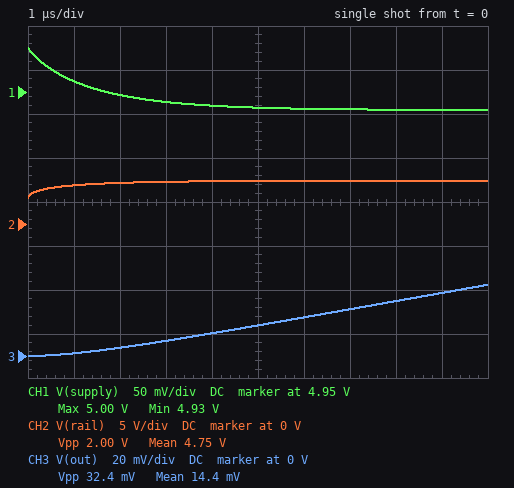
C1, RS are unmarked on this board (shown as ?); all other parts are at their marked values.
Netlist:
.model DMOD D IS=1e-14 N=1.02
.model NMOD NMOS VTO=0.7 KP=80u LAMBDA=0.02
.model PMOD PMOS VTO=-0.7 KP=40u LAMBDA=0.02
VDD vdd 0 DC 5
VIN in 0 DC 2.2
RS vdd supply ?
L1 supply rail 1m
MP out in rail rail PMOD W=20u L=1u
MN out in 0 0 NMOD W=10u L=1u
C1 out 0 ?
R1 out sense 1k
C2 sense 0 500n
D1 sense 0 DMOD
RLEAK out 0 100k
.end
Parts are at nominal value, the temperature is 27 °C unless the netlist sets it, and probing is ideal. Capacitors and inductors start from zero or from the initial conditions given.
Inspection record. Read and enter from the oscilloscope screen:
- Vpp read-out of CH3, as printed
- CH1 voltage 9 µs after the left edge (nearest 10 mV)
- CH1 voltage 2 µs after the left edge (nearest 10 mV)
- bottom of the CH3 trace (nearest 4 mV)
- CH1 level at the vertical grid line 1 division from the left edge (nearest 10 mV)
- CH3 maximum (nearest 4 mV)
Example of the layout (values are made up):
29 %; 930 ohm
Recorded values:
32.4 mV; 4.93 V; 4.95 V; 0 V; 4.96 V; 32 mV
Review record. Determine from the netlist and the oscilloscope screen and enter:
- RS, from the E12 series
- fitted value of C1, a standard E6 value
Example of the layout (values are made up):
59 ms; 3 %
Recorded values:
39 Ω; 470 nF
